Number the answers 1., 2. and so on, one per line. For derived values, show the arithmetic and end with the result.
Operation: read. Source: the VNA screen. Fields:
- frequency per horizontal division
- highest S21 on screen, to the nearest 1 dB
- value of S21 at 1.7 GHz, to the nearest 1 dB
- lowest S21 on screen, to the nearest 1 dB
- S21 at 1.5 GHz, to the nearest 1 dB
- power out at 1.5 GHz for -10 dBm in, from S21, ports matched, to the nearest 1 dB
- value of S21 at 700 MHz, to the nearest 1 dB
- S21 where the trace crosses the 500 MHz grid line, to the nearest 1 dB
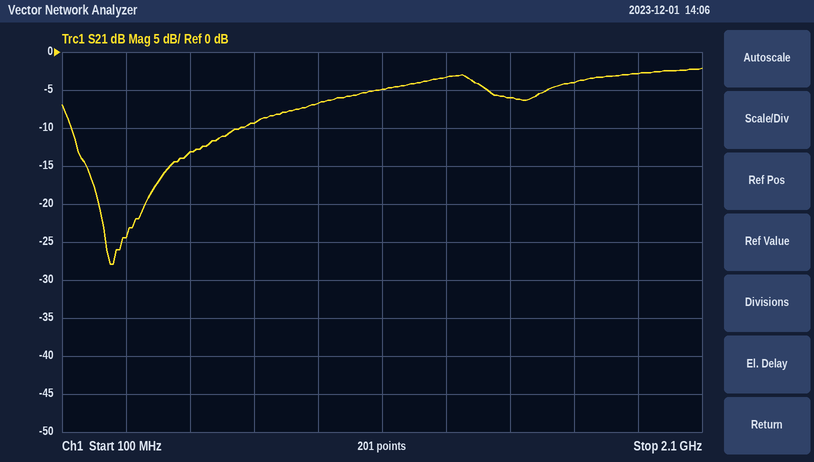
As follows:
1. 200 MHz
2. -2 dB
3. -4 dB
4. -28 dB
5. -6 dB
6. -10 dBm + (-6 dB) = -16 dBm
7. -9 dB
8. -13 dB
